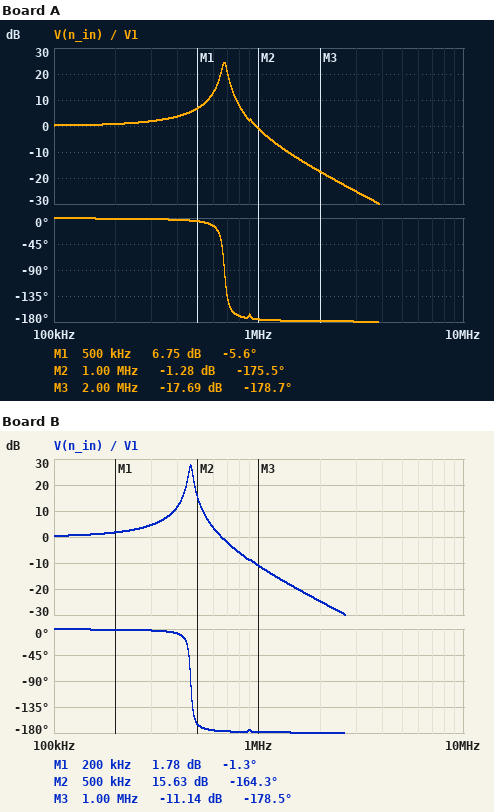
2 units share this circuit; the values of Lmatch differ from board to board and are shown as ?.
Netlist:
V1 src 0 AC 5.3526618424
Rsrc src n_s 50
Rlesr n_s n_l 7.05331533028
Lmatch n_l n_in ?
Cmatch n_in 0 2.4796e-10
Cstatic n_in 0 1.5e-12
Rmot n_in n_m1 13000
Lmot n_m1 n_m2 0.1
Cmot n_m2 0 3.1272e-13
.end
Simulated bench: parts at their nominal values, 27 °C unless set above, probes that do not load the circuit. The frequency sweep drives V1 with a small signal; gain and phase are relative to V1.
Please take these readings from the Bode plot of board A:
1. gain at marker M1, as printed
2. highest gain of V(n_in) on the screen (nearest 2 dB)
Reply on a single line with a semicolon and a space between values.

6.75 dB; 24 dB
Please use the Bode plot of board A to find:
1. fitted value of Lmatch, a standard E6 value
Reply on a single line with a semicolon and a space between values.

220 µH
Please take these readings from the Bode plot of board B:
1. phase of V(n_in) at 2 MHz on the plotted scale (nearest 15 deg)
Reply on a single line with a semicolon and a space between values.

-180 deg
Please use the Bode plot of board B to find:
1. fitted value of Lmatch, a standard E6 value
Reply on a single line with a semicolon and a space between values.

470 µH
